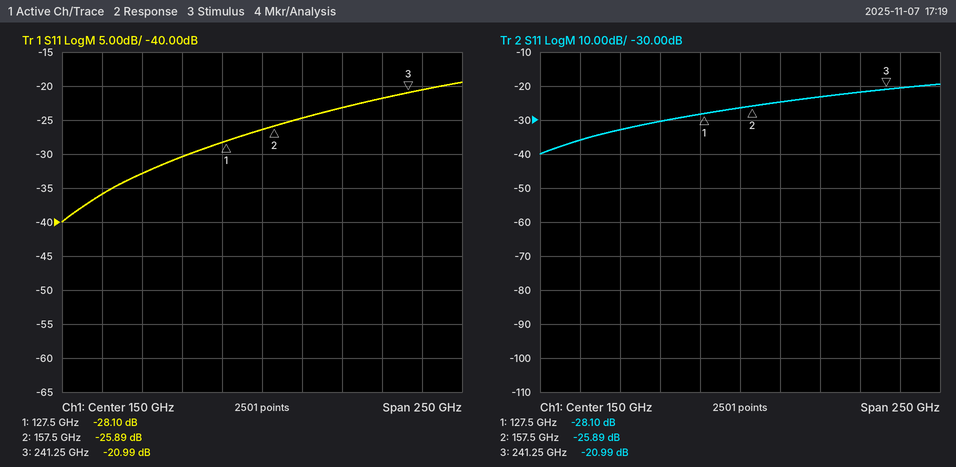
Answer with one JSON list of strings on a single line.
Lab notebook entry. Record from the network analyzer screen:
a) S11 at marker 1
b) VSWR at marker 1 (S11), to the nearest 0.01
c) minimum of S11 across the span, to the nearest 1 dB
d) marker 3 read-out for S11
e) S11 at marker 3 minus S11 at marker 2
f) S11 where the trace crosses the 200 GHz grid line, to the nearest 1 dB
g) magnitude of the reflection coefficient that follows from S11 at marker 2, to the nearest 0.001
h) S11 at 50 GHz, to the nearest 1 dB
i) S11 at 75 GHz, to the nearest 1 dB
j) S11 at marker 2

["-28.10 dB", "1.08", "-40 dB", "-20.99 dB", "4.90 dB", "-23 dB", "0.051", "-36 dB", "-33 dB", "-25.89 dB"]
